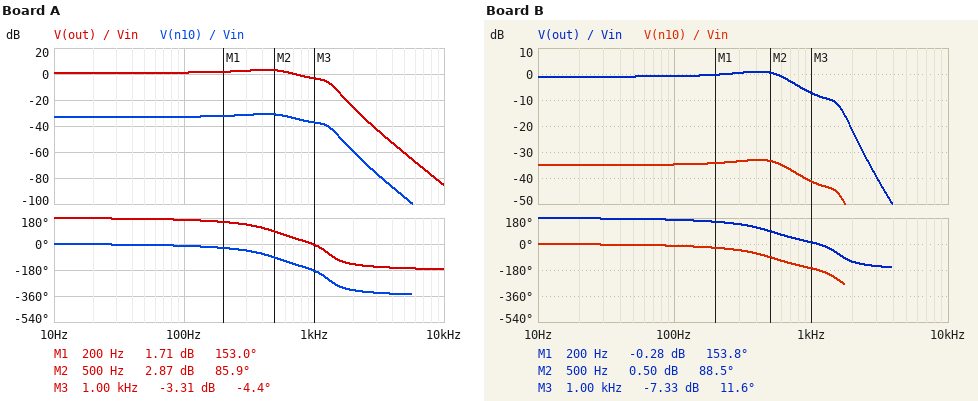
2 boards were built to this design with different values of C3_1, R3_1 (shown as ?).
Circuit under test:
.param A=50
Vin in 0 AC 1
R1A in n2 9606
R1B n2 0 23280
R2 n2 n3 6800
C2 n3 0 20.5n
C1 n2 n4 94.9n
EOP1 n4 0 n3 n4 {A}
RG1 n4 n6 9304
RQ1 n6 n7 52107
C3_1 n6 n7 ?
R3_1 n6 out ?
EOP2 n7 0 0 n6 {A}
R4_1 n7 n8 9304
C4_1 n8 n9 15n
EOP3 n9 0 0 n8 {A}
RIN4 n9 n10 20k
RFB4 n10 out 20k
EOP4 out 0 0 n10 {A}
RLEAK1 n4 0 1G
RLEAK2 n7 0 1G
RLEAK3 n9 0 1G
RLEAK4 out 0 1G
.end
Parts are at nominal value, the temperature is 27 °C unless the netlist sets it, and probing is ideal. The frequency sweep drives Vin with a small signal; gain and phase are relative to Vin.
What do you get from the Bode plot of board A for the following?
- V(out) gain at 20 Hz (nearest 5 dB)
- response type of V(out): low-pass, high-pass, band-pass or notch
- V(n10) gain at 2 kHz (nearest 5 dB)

0 dB
low-pass
-60 dB
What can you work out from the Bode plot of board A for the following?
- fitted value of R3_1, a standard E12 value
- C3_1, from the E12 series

15 kΩ
6.8 nF
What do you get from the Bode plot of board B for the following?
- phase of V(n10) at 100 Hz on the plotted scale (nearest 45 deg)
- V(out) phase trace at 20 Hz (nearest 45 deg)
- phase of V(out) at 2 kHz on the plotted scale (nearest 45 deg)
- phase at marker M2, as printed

0 deg
180 deg
-135 deg
88.5 deg
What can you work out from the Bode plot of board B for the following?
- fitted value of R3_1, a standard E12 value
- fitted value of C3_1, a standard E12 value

12 kΩ
5.6 nF
